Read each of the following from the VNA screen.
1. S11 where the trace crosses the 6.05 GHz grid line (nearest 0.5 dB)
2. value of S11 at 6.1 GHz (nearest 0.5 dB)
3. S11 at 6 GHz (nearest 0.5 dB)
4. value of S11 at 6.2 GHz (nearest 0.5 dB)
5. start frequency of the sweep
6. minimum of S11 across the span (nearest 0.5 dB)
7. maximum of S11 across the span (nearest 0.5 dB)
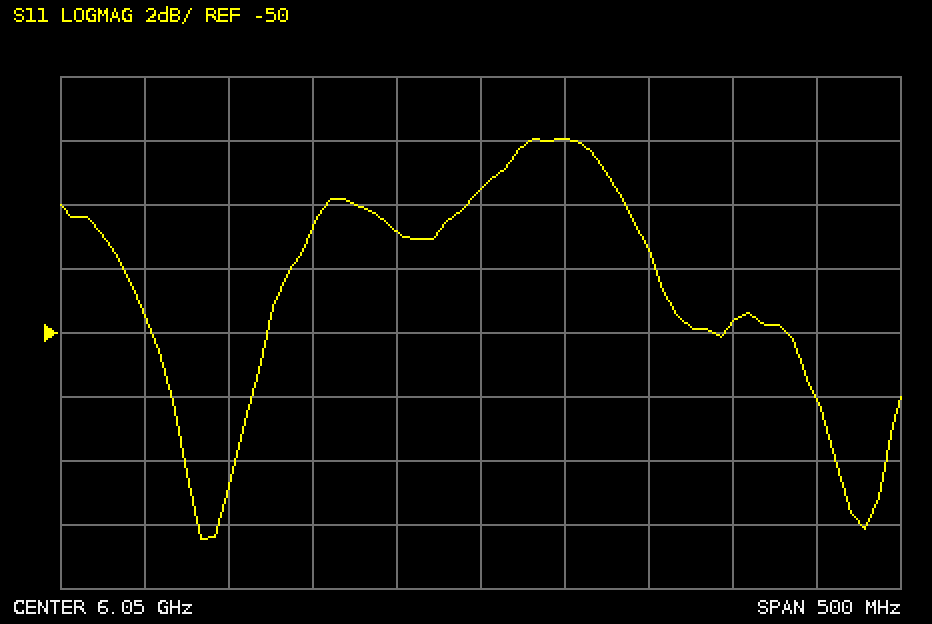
-45.5 dB
-44.0 dB
-47.0 dB
-49.5 dB
5.8 GHz
-56.5 dB
-44.0 dB
